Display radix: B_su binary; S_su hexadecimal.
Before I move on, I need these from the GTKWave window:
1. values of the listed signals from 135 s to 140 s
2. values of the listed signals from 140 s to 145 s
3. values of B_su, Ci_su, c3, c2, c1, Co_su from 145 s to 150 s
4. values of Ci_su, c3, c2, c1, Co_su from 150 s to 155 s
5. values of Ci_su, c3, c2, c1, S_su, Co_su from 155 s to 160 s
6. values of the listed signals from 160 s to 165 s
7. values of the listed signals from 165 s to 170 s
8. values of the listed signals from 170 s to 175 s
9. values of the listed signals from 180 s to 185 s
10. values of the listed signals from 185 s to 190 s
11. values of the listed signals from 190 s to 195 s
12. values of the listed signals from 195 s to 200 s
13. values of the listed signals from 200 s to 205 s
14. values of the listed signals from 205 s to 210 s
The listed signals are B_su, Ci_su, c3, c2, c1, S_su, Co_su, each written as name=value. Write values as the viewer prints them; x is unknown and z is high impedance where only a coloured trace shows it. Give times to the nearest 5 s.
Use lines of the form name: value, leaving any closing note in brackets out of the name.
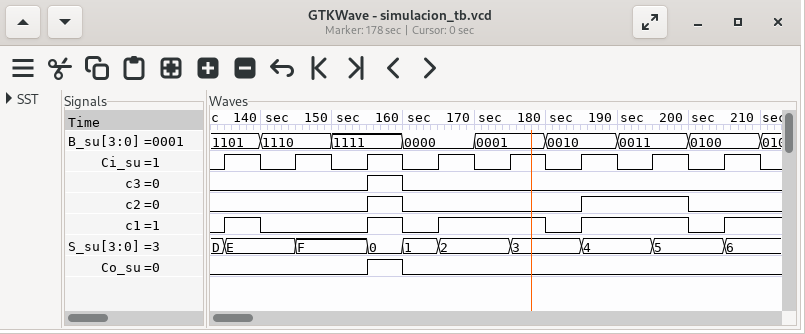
values of the listed signals from 135 s to 140 s: B_su=1101, Ci_su=1, c3=0, c2=0, c1=1, S_su=E, Co_su=0
values of the listed signals from 140 s to 145 s: B_su=1110, Ci_su=0, c3=0, c2=0, c1=0, S_su=E, Co_su=0
values of B_su, Ci_su, c3, c2, c1, Co_su from 145 s to 150 s: B_su=1110, Ci_su=1, c3=0, c2=0, c1=0, Co_su=0
values of Ci_su, c3, c2, c1, Co_su from 150 s to 155 s: Ci_su=0, c3=0, c2=0, c1=0, Co_su=0
values of Ci_su, c3, c2, c1, S_su, Co_su from 155 s to 160 s: Ci_su=1, c3=1, c2=1, c1=1, S_su=0, Co_su=1
values of the listed signals from 160 s to 165 s: B_su=0000, Ci_su=0, c3=0, c2=0, c1=0, S_su=1, Co_su=0
values of the listed signals from 165 s to 170 s: B_su=0000, Ci_su=1, c3=0, c2=0, c1=1, S_su=2, Co_su=0
values of the listed signals from 170 s to 175 s: B_su=0001, Ci_su=0, c3=0, c2=0, c1=1, S_su=2, Co_su=0
values of the listed signals from 180 s to 185 s: B_su=0010, Ci_su=0, c3=0, c2=0, c1=0, S_su=3, Co_su=0
values of the listed signals from 185 s to 190 s: B_su=0010, Ci_su=1, c3=0, c2=1, c1=1, S_su=4, Co_su=0
values of the listed signals from 190 s to 195 s: B_su=0011, Ci_su=0, c3=0, c2=1, c1=1, S_su=4, Co_su=0
values of the listed signals from 195 s to 200 s: B_su=0011, Ci_su=1, c3=0, c2=1, c1=1, S_su=5, Co_su=0
values of the listed signals from 200 s to 205 s: B_su=0100, Ci_su=0, c3=0, c2=0, c1=0, S_su=5, Co_su=0
values of the listed signals from 205 s to 210 s: B_su=0100, Ci_su=1, c3=0, c2=0, c1=1, S_su=6, Co_su=0
